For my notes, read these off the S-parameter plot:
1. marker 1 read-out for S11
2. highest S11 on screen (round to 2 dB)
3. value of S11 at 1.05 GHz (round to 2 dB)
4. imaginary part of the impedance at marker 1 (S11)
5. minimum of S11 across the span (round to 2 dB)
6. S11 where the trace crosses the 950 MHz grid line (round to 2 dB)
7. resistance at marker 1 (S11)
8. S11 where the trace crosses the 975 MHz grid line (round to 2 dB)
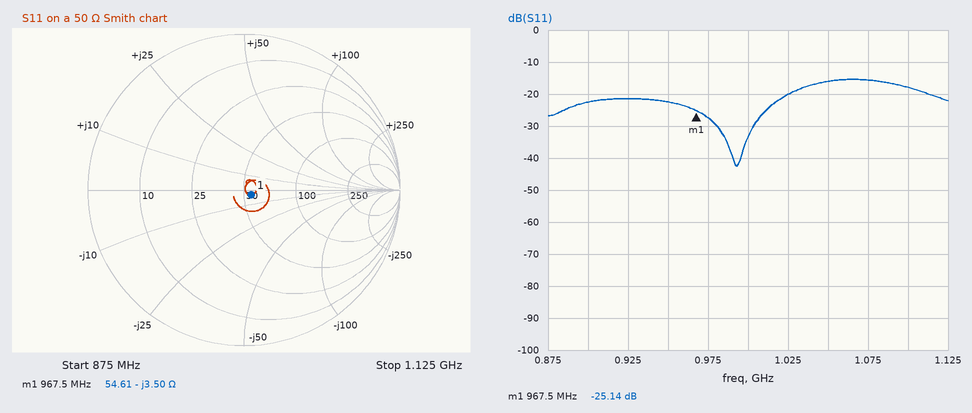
-25.14 dB
-16 dB
-16 dB
-3.50 Ω
-42 dB
-22 dB
54.61 Ω
-28 dB
